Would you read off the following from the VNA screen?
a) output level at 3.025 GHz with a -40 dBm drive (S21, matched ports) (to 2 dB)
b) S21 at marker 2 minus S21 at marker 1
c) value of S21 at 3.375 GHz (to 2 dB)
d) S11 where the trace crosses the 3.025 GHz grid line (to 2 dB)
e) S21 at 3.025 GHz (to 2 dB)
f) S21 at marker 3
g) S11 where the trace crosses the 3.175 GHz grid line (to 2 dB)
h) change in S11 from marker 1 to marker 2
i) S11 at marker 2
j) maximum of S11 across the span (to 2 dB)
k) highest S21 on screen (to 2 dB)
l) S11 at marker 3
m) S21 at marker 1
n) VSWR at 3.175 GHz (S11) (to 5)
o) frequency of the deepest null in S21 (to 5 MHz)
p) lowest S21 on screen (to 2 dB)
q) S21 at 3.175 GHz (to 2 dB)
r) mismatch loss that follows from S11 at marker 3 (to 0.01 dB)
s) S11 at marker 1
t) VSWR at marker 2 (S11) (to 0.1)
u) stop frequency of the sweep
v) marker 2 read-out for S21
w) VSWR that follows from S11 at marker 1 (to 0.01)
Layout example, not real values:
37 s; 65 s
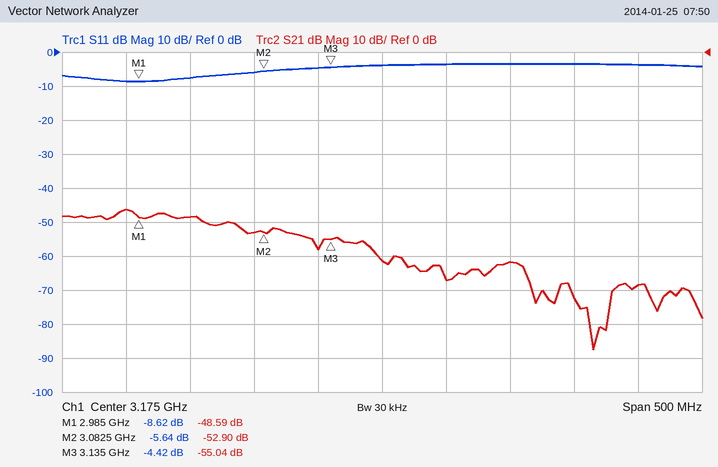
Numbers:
-88 dBm; -4.31 dB; -68 dB; -8 dB; -48 dB; -55.04 dB; -4 dB; 2.98 dB; -5.64 dB; -4 dB; -46 dB; -4.42 dB; -48.59 dB; 5; 3.340 GHz; -88 dB; -62 dB; 1.95 dB; -8.62 dB; 3.2; 3.425 GHz; -52.90 dB; 2.18
